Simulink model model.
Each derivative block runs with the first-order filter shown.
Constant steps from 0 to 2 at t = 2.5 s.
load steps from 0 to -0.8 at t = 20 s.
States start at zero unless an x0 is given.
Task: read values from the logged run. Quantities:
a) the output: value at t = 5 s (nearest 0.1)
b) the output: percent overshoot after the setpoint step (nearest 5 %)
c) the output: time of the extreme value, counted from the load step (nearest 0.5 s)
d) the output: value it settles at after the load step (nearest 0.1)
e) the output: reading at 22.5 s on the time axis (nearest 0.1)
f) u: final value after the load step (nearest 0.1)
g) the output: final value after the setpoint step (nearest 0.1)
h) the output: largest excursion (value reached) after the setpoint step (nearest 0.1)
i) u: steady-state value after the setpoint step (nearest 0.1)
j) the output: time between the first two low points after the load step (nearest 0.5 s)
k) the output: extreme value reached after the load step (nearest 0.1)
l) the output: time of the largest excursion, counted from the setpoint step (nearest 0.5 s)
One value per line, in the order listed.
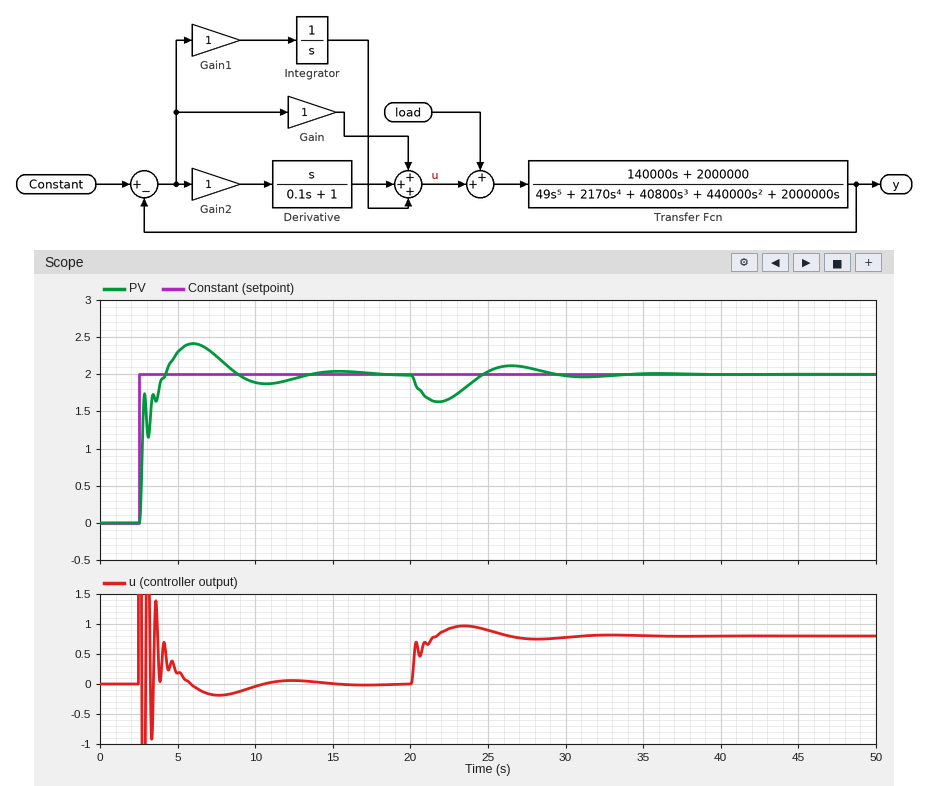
2.3
20 %
2.0 s
2.0
1.7
0.8
2.0
2.4
0.0
9.5 s
1.6
3.5 s
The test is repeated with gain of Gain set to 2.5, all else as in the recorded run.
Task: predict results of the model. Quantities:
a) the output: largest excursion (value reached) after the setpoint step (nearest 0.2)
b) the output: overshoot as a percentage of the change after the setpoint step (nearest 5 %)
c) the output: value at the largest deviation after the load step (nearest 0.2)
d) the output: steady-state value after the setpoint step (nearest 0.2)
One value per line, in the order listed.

2.2
10 %
1.8
2.0
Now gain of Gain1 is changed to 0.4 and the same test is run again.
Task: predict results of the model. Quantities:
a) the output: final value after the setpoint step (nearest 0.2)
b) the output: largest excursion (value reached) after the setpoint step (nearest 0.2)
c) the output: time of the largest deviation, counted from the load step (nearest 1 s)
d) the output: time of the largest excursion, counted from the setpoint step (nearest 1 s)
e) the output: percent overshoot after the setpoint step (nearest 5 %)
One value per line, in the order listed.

2.0
2.2
3 s
5 s
15 %
